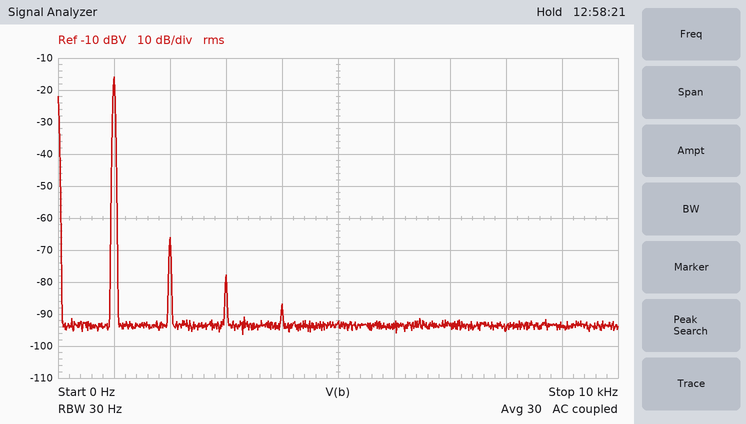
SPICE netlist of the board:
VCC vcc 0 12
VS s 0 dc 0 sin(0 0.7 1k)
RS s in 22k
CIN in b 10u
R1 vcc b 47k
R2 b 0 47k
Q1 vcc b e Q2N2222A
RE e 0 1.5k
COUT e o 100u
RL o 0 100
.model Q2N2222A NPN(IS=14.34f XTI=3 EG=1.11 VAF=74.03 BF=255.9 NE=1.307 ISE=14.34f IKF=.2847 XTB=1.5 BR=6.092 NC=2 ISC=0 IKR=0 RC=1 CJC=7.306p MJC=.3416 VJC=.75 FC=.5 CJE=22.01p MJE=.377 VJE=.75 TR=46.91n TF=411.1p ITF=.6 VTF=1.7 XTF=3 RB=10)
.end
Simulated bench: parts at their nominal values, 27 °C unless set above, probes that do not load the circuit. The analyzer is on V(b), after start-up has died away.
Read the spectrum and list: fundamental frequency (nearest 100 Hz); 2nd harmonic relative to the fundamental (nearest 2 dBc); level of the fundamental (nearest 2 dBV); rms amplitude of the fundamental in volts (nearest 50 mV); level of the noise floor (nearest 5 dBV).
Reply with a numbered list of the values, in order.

1. 1.0 kHz
2. -50 dBc
3. -16 dBV
4. 150 mV
5. -95 dBV
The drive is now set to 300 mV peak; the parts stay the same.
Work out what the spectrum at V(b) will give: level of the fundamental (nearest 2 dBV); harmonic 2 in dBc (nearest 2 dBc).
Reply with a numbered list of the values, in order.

1. -24 dBV
2. -60 dBc
